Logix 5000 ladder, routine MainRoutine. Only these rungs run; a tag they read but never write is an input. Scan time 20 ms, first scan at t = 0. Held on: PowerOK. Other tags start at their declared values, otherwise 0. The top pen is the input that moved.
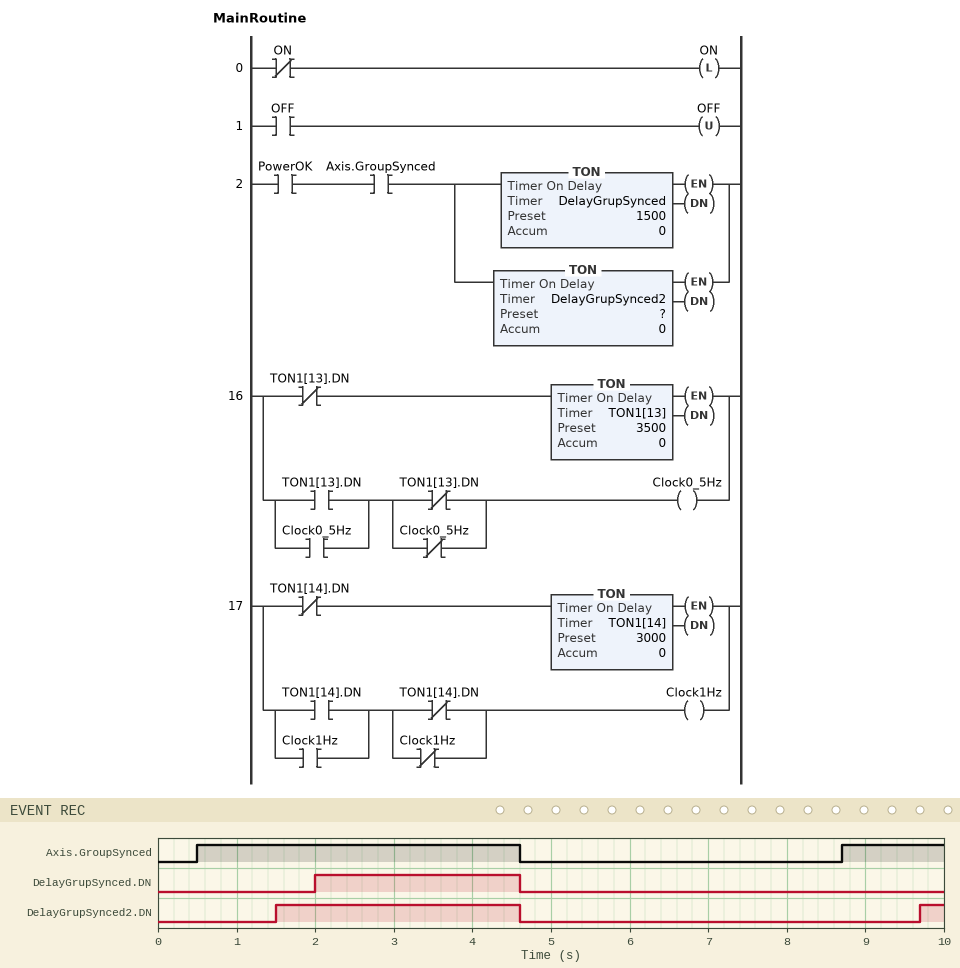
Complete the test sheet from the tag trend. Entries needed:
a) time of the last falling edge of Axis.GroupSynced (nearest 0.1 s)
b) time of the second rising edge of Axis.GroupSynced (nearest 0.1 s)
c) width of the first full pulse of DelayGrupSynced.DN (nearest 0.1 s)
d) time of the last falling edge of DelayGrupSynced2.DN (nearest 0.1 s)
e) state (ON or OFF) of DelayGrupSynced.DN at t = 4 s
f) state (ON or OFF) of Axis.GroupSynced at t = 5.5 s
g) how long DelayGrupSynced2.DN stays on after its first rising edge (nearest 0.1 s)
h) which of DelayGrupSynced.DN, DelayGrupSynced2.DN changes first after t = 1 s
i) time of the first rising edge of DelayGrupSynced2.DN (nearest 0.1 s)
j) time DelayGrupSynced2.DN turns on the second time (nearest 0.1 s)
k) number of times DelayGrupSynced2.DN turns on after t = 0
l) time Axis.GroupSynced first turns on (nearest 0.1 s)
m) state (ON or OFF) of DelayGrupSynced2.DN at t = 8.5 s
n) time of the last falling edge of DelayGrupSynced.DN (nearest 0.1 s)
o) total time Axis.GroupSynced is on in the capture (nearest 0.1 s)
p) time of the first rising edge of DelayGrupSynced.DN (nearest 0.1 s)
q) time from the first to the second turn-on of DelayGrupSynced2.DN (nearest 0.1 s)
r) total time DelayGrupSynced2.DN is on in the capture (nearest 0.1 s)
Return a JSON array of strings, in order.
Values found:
["4.6 s", "8.7 s", "2.6 s", "4.6 s", "ON", "OFF", "3.1 s", "DelayGrupSynced2.DN", "1.5 s", "9.7 s", "2", "0.5 s", "OFF", "4.6 s", "5.4 s", "2.0 s", "8.2 s", "3.4 s"]
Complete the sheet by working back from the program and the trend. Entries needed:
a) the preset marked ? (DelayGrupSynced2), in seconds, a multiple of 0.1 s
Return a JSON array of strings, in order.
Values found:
["1.0 s"]
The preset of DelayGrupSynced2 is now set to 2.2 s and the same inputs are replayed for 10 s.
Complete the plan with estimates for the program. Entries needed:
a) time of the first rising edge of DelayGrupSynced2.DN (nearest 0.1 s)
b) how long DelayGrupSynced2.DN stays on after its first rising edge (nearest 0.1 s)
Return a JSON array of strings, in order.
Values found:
["2.7 s", "1.9 s"]
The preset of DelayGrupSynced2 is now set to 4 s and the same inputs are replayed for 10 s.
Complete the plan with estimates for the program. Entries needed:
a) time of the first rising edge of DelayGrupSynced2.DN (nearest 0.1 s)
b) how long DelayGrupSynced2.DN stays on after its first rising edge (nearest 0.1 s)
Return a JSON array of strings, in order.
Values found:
["4.5 s", "0.1 s"]
